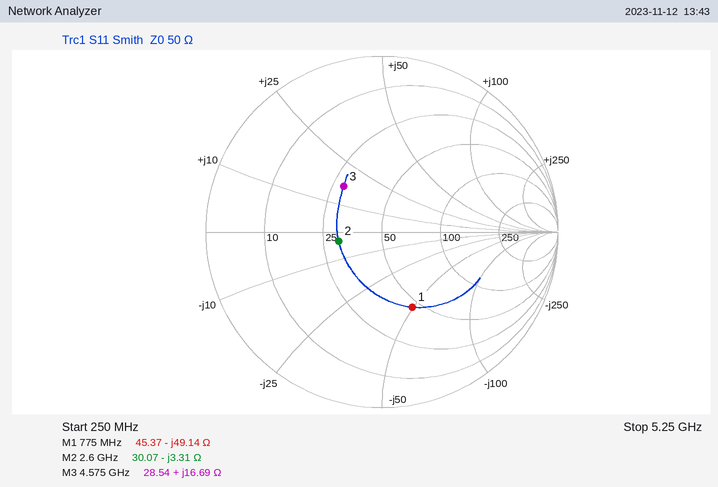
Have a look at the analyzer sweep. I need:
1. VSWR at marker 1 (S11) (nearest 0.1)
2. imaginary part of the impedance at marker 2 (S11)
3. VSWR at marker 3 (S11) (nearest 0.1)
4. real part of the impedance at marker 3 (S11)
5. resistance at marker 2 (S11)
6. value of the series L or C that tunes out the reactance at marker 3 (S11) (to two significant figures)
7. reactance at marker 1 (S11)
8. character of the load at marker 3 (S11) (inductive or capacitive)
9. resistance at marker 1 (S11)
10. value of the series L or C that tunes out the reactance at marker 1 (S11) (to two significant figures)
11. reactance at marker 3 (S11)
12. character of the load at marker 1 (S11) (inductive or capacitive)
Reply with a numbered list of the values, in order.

1. 2.7
2. -3.31 Ω
3. 2.0
4. 28.54 Ω
5. 30.07 Ω
6. 2.1 pF
7. -49.14 Ω
8. inductive
9. 45.37 Ω
10. 10 nH
11. +16.69 Ω
12. capacitive
